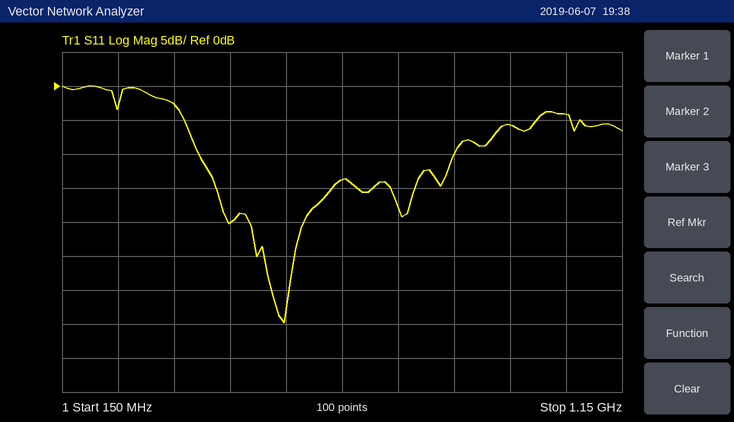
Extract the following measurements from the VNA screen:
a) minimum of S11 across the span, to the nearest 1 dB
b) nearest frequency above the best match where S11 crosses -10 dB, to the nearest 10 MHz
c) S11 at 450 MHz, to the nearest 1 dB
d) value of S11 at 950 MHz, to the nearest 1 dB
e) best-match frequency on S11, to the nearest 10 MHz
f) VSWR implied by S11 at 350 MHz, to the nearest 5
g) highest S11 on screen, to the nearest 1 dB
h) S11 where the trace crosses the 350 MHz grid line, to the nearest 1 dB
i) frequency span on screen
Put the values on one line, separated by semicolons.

-35 dB; 850 MHz; -20 dB; -6 dB; 550 MHz; 5; 0 dB; -3 dB; 1 GHz
